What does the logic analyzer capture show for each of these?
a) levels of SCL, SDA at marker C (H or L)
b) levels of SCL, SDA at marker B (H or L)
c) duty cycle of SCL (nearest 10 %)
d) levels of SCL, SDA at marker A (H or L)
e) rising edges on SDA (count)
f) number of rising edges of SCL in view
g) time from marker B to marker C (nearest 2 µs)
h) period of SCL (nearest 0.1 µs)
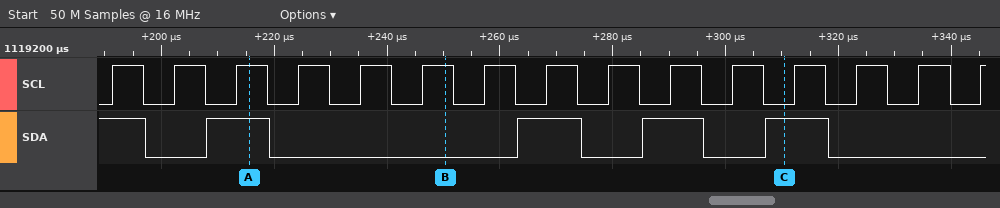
SCL=L, SDA=H
SCL=H, SDA=L
50 %
SCL=H, SDA=H
4
15
60 µs
11 µs
